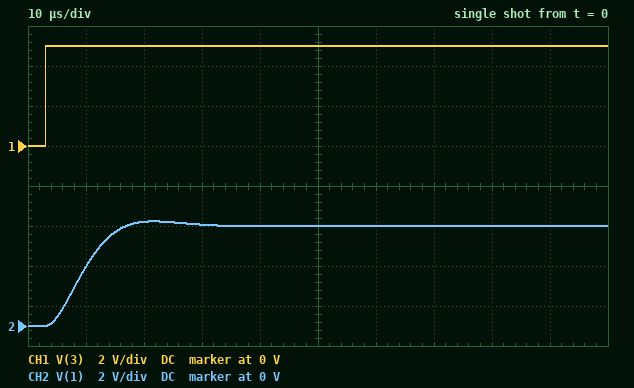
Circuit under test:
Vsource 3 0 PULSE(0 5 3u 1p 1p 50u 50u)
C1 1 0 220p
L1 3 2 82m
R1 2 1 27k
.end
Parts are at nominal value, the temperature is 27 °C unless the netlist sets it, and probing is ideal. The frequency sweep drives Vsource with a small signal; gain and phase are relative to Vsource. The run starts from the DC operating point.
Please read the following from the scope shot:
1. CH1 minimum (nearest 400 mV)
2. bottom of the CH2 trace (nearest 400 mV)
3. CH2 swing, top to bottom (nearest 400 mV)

0 V
0 V
5.2 V
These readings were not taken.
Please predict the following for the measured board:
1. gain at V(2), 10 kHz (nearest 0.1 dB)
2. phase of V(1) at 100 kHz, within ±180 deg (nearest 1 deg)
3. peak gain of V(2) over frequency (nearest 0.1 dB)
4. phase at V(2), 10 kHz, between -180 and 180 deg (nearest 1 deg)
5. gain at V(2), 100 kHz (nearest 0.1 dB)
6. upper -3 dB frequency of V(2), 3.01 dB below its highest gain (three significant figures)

0.6 dB
-149 deg
2.1 dB
-1 deg
-5.4 dB
59.6 kHz
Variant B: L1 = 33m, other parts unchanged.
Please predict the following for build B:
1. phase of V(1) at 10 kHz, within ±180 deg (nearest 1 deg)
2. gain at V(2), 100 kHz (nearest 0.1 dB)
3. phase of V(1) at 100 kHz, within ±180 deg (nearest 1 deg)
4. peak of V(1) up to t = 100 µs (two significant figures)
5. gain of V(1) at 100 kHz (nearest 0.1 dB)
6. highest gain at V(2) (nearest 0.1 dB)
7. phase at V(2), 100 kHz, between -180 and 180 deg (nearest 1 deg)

-21 deg
-0.7 dB
-117 deg
5.0 V
-12.4 dB
1.1 dB
-42 deg
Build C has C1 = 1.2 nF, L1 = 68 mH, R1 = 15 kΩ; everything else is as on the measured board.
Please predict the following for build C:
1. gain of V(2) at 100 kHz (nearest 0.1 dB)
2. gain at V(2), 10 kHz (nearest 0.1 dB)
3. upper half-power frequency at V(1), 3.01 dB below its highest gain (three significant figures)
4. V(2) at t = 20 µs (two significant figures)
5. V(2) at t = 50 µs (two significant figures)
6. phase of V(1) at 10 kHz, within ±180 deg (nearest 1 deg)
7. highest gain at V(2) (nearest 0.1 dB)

-9.3 dB
1.2 dB
11.4 kHz
5.7 V
5.1 V
-59 deg
1.3 dB
